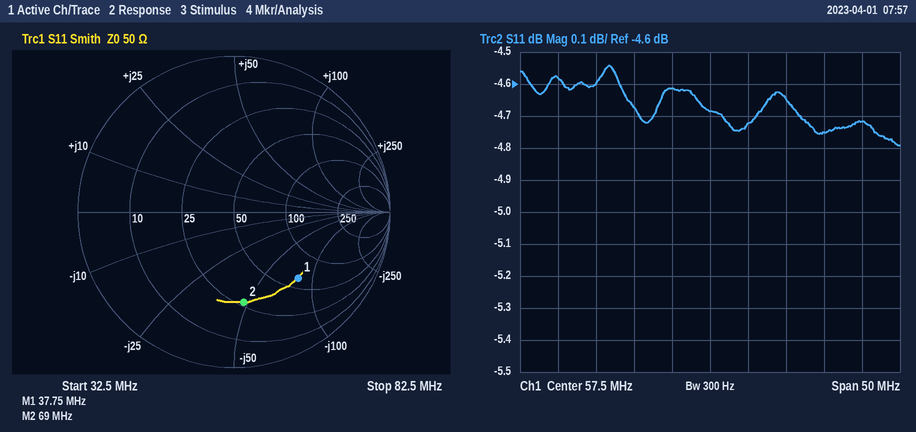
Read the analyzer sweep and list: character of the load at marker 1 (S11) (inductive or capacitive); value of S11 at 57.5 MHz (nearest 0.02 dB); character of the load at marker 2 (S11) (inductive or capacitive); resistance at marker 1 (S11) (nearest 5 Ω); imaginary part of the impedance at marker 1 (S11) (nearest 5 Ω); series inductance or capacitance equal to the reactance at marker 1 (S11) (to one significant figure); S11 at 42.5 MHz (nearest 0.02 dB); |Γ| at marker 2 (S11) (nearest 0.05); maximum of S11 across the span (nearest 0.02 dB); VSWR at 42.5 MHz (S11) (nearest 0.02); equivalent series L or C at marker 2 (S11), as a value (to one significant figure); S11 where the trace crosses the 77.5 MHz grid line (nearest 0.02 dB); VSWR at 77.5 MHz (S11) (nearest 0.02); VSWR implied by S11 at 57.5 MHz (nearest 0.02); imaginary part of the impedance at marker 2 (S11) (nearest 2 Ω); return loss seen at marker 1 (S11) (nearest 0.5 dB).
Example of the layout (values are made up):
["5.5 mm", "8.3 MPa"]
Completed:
["capacitive", "-4.68 dB", "capacitive", "60 Ω", "-80 Ω", "50 pF", "-4.60 dB", "0.60", "-4.54 dB", "3.86", "50 pF", "-4.72 dB", "3.78", "3.80", "-48 Ω", "4.5 dB"]
